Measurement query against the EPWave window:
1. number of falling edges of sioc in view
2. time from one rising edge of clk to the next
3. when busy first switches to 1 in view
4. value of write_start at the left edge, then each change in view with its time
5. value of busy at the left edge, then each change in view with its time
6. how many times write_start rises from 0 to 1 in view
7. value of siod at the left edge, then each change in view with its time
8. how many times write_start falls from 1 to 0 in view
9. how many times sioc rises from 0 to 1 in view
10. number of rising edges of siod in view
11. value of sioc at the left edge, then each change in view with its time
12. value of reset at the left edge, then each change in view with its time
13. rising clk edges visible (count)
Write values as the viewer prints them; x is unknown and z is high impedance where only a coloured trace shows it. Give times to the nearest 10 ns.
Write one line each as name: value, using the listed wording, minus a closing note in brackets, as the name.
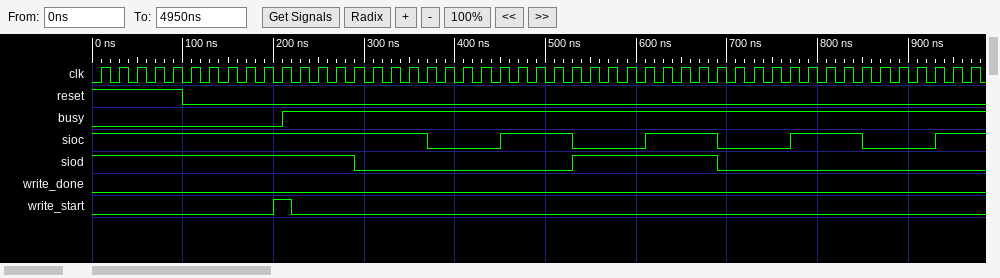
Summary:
number of falling edges of sioc in view: 4
time from one rising edge of clk to the next: 20 ns
when busy first switches to 1 in view: 210 ns
value of write_start at the left edge, then each change in view with its time: 0, 1 at 200 ns, 0 at 220 ns
value of busy at the left edge, then each change in view with its time: 0, 1 at 210 ns
how many times write_start rises from 0 to 1 in view: 1
value of siod at the left edge, then each change in view with its time: 1, 0 at 290 ns, 1 at 530 ns, 0 at 690 ns
how many times write_start falls from 1 to 0 in view: 1
how many times sioc rises from 0 to 1 in view: 4
number of rising edges of siod in view: 1
value of sioc at the left edge, then each change in view with its time: 1, 0 at 370 ns, 1 at 450 ns, 0 at 530 ns, 1 at 610 ns, 0 at 690 ns, 1 at 770 ns, 0 at 850 ns, 1 at 930 ns
value of reset at the left edge, then each change in view with its time: 1, 0 at 100 ns
rising clk edges visible: 49
